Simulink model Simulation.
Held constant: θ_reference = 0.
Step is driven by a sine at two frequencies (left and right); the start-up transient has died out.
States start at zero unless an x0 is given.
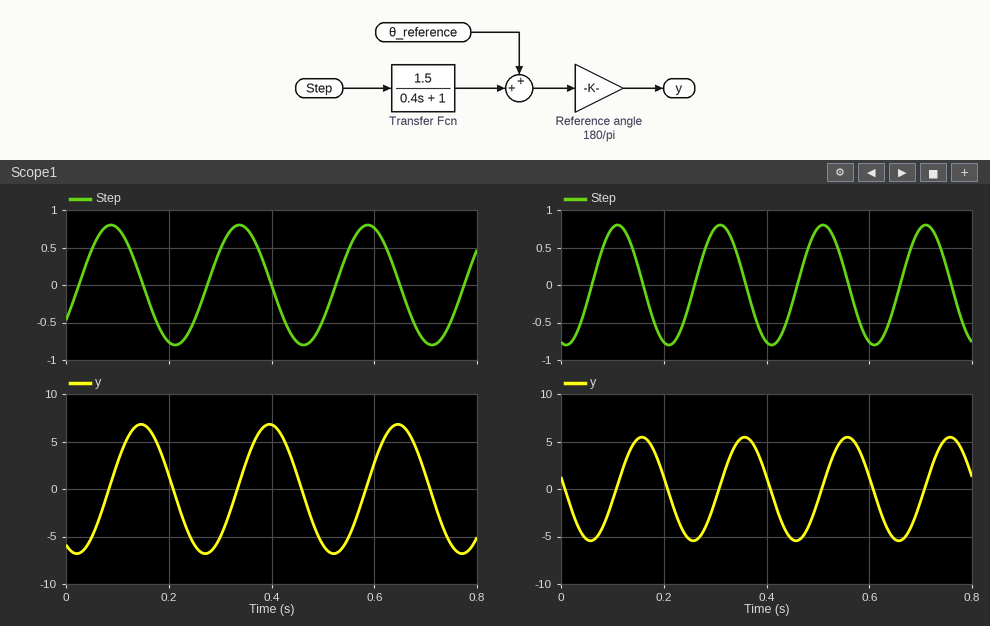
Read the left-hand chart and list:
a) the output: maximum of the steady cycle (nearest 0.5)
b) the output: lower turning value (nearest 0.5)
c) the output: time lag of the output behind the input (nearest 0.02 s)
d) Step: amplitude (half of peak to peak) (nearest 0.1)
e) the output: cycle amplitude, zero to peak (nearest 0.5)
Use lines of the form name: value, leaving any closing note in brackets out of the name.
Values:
the output: maximum of the steady cycle: 7.0
the output: lower turning value: -7.0
the output: time lag of the output behind the input: 0.06 s
Step: amplitude (half of peak to peak): 0.8
the output: cycle amplitude, zero to peak: 7.0
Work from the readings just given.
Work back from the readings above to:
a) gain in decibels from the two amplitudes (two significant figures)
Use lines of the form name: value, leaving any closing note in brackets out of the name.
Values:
gain in decibels from the two amplitudes: 19 dB
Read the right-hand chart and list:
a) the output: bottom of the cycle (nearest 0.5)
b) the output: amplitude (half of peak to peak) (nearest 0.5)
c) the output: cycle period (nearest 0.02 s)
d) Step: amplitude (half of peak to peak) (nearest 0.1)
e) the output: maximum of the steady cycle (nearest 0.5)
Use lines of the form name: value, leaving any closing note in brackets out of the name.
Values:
the output: bottom of the cycle: -5.5
the output: amplitude (half of peak to peak): 5.5
the output: cycle period: 0.20 s
Step: amplitude (half of peak to peak): 0.8
the output: maximum of the steady cycle: 5.5
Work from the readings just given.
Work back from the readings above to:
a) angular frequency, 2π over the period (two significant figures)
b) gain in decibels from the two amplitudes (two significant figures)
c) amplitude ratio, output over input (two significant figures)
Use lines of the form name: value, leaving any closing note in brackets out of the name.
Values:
angular frequency, 2π over the period: 31 rad/s
gain in decibels from the two amplitudes: 17 dB
amplitude ratio, output over input: 6.9
